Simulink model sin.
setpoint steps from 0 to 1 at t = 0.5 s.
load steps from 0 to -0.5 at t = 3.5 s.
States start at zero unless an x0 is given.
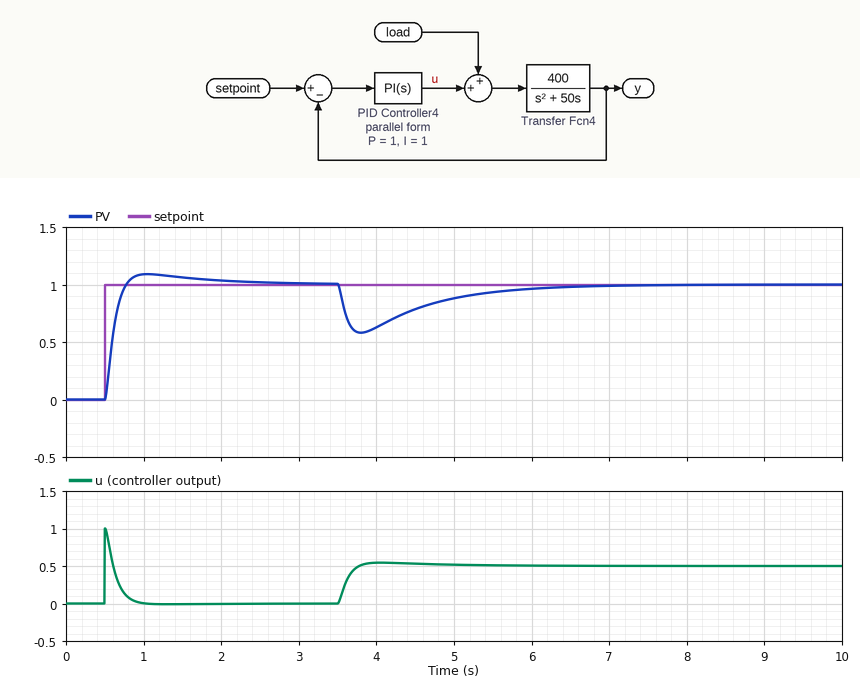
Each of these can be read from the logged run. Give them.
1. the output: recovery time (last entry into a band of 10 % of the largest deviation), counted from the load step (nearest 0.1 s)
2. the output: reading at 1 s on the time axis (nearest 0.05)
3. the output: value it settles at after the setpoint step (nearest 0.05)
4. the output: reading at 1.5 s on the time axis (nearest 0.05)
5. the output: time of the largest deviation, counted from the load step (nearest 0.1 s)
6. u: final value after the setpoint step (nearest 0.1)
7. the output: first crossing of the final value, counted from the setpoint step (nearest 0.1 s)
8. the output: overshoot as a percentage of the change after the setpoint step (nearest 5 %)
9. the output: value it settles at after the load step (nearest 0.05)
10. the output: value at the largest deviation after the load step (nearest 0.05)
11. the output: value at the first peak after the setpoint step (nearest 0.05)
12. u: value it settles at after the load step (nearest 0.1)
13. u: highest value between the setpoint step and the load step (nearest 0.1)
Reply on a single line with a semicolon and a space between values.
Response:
2.4 s; 1.10; 1.00; 1.05; 0.3 s; 0.0; 0.3 s; 10 %; 1.00; 0.60; 1.10; 0.5; 1.0
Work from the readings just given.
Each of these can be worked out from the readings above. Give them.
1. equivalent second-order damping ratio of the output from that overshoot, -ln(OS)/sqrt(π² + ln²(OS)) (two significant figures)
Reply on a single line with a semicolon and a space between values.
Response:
0.59
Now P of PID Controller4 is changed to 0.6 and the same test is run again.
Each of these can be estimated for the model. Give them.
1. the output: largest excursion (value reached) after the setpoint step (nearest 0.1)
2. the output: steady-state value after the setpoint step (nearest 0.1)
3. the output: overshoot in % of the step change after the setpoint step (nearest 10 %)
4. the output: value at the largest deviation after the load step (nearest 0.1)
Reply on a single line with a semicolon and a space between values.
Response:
1.2; 1.0; 20 %; 0.4
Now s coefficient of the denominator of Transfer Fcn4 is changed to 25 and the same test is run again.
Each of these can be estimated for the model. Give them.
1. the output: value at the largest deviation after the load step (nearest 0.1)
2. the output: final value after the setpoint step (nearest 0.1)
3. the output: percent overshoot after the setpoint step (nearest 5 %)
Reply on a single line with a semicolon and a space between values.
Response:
0.5; 1.0; 15 %
